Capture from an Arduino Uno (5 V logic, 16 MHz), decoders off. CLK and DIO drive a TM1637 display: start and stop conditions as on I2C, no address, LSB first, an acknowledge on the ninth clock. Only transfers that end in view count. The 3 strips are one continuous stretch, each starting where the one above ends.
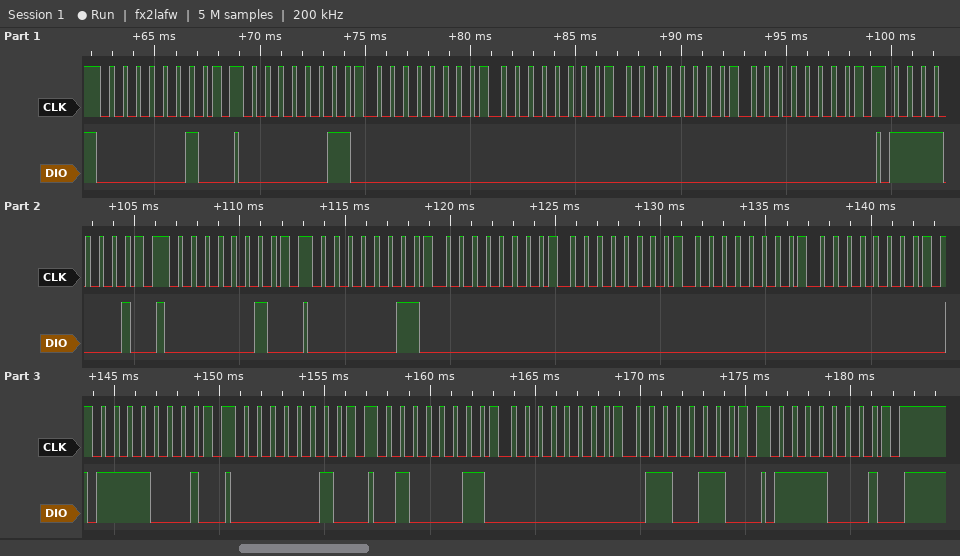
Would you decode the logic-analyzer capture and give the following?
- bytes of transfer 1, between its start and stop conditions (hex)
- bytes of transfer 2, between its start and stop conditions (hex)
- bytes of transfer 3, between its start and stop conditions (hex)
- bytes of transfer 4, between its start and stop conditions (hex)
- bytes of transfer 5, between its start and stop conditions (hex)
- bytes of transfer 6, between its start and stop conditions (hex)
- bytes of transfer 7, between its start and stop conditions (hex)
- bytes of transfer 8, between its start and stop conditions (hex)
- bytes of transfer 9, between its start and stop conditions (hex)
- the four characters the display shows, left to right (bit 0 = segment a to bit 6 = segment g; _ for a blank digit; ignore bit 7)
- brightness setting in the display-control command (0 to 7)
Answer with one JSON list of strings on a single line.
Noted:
["40", "C0 00 00 00 00", "8F", "40", "C0 00 00 00 00", "8F", "40", "C2 00 66", "8F", "___4", "7"]
